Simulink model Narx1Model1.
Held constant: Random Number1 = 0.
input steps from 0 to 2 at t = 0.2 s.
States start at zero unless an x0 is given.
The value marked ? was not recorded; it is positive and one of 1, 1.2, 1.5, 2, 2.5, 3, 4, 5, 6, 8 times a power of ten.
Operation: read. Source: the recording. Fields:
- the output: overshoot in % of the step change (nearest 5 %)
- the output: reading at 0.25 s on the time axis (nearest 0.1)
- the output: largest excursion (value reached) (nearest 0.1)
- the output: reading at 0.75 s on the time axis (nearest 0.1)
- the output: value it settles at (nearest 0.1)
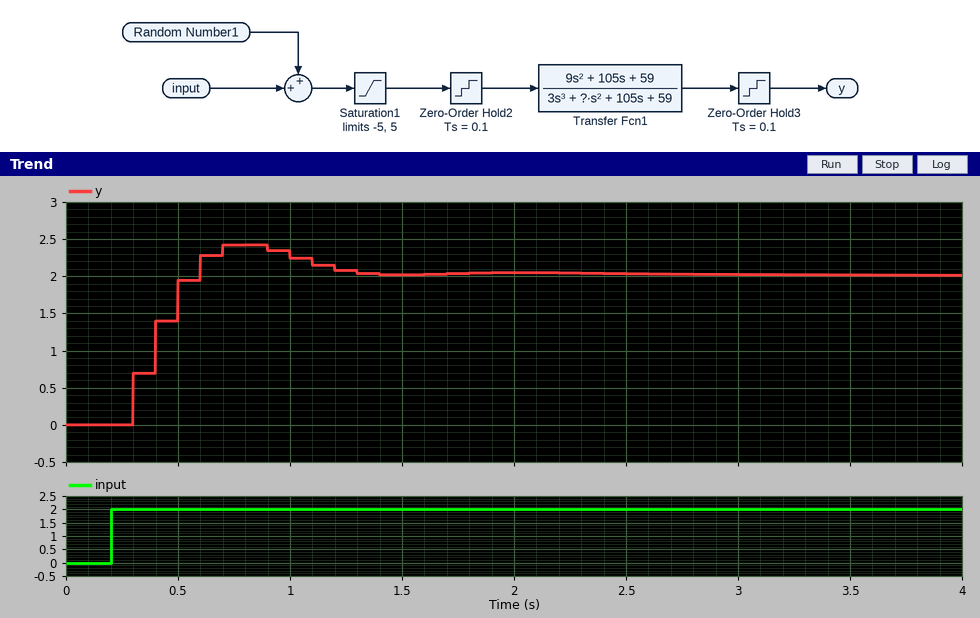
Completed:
20 %
0.0
2.4
2.4
2.0
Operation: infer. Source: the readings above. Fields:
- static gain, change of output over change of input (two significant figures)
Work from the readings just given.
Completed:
1.0
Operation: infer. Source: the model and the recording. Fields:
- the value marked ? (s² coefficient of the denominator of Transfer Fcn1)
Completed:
20
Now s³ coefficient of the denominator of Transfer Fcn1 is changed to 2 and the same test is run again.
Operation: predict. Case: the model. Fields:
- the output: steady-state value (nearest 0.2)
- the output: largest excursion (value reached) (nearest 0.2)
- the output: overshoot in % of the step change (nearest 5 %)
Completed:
2.0
2.2
15 %
